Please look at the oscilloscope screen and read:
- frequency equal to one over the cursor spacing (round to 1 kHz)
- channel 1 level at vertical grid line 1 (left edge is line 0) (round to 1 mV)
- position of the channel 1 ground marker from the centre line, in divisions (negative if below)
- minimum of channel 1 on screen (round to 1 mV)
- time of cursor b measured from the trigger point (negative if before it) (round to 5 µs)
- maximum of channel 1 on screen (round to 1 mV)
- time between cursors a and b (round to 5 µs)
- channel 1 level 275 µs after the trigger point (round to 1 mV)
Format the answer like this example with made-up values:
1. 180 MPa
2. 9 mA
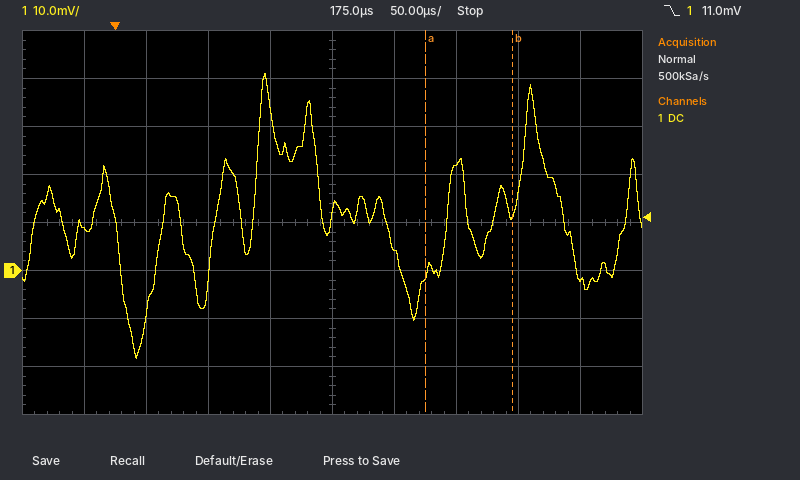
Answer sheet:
1. 14 kHz
2. 9 mV
3. -1.0 div
4. -18 mV
5. +320 µs
6. 41 mV
7. 70 µs
8. 22 mV
